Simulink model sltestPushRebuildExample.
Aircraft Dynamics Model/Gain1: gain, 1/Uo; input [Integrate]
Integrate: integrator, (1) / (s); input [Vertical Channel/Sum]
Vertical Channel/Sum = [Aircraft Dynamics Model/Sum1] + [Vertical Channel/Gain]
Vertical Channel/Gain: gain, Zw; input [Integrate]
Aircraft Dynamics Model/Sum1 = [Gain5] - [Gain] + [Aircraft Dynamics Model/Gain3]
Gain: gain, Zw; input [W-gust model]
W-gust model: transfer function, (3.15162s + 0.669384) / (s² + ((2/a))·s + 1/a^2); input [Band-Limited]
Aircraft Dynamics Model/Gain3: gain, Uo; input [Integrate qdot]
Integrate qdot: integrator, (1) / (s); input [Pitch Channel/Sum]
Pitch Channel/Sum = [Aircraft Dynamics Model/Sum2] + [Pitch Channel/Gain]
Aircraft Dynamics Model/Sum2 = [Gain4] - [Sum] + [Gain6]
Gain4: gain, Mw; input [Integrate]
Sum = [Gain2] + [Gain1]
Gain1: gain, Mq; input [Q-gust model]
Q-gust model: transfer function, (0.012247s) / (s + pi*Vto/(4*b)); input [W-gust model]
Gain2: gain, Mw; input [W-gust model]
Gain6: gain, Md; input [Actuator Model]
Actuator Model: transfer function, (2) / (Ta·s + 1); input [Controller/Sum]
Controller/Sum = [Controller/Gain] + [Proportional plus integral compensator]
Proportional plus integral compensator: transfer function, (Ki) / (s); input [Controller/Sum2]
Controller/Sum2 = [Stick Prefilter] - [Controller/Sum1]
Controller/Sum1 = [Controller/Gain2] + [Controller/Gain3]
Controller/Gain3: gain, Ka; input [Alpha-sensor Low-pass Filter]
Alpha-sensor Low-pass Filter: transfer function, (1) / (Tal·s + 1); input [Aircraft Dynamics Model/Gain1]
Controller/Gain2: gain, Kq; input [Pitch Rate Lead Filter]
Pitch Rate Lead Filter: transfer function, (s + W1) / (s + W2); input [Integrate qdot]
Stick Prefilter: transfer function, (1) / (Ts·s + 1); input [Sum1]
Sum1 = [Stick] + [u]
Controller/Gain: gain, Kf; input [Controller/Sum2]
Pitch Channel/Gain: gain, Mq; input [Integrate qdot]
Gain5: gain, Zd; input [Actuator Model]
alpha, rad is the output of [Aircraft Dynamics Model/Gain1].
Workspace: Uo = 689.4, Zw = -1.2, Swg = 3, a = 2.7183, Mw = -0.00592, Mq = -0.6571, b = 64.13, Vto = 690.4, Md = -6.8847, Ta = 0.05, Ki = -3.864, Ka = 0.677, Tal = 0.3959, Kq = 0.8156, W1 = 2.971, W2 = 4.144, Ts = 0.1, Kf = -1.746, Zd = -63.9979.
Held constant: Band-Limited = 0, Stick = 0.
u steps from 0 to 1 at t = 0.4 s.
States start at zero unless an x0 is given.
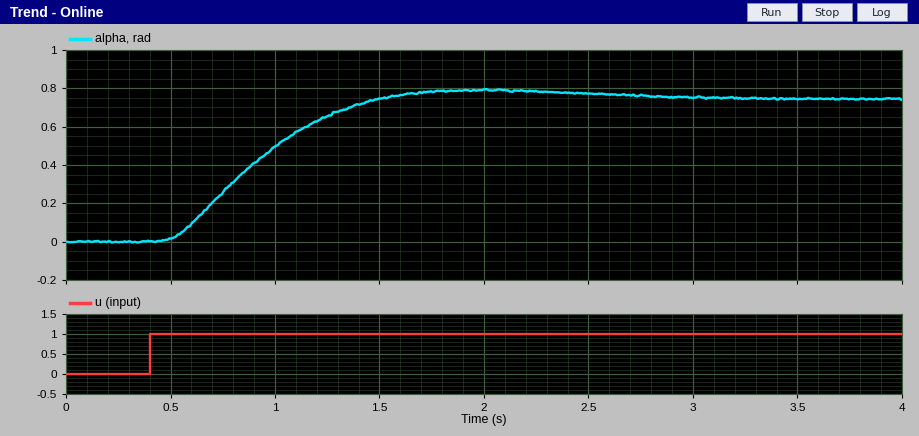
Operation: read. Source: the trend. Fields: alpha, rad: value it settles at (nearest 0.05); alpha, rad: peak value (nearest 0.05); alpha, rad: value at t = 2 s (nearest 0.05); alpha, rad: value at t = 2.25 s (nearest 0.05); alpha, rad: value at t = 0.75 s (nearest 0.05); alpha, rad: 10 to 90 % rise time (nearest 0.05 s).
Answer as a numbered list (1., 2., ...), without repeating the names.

1. 0.75
2. 0.80
3. 0.80
4. 0.80
5. 0.25
6. 0.70 s
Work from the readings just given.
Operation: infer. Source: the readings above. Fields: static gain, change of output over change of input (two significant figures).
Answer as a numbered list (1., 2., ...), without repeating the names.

1. 0.75
